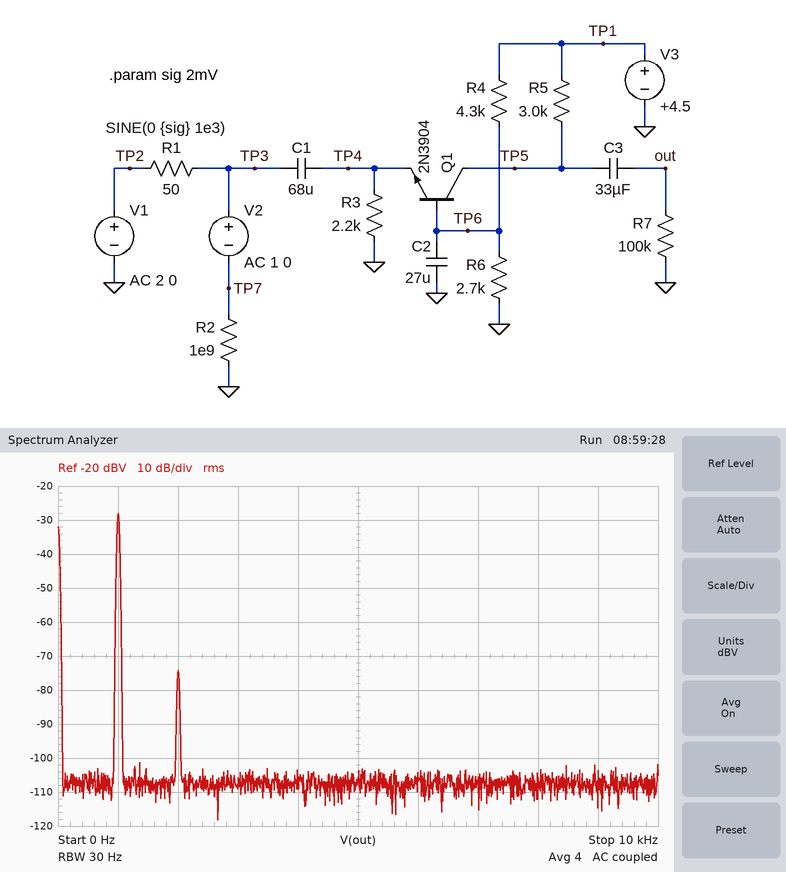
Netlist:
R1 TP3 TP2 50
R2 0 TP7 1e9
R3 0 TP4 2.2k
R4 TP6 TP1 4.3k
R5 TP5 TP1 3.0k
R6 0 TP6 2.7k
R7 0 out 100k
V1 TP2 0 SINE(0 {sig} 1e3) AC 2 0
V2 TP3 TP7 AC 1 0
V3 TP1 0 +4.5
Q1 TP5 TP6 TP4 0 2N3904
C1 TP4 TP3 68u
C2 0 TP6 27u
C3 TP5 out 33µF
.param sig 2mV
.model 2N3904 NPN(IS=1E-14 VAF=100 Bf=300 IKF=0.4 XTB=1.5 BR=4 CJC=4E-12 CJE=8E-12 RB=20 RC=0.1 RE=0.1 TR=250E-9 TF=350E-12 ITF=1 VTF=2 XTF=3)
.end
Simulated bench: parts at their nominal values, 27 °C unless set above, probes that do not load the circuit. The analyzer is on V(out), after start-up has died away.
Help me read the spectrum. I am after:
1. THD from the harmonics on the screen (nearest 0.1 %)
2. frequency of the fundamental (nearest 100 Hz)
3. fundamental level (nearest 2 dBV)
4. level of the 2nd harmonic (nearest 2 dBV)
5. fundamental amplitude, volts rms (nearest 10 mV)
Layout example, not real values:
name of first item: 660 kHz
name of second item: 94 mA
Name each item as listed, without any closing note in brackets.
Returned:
THD from the harmonics on the screen: 0.5 %
frequency of the fundamental: 1.0 kHz
fundamental level: -28 dBV
level of the 2nd harmonic: -74 dBV
fundamental amplitude, volts rms: 40 mV
